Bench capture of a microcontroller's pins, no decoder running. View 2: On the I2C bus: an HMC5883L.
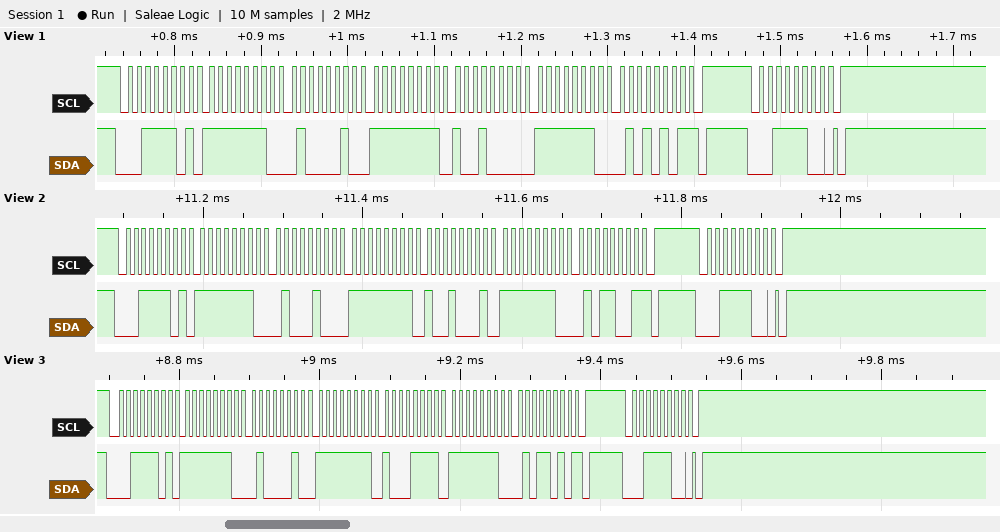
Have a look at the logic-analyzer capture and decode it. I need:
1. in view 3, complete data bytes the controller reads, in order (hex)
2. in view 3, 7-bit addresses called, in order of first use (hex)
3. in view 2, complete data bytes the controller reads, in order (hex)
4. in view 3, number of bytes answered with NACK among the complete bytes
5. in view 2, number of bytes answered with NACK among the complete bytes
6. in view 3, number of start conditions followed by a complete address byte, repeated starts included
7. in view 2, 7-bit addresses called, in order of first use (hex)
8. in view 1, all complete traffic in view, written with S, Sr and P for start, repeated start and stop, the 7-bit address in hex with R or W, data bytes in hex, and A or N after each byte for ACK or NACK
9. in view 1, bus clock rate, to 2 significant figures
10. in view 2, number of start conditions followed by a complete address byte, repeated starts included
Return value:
FE 42 FF 8F FE 5A
0x1E
FE 44 FF 91 FE 59
1
1
2
0x1E
S 1ER A FE A 42 A FF A 90 A FE A 55 N P S 1EW A P
100 kHz
2
